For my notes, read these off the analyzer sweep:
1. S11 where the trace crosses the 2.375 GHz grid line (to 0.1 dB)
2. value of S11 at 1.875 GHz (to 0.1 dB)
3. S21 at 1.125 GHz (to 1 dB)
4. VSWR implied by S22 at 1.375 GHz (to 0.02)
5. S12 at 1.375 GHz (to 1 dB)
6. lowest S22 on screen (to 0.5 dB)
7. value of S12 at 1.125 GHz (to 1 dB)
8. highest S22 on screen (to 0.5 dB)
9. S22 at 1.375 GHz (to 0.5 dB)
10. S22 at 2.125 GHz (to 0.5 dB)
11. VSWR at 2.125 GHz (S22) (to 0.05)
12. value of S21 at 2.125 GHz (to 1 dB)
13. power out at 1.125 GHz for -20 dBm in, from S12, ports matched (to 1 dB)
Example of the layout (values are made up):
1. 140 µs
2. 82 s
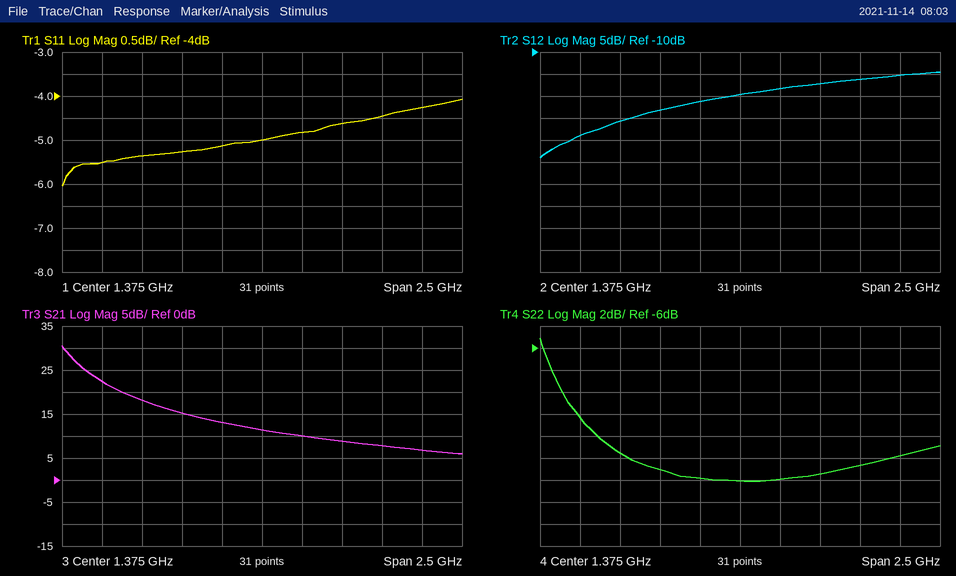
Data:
1. -4.3 dB
2. -4.6 dB
3. 13 dB
4. 1.28
5. -20 dB
6. -18.0 dB
7. -21 dB
8. -5.0 dB
9. -18.0 dB
10. -16.5 dB
11. 1.35
12. 8 dB
13. -41 dBm
